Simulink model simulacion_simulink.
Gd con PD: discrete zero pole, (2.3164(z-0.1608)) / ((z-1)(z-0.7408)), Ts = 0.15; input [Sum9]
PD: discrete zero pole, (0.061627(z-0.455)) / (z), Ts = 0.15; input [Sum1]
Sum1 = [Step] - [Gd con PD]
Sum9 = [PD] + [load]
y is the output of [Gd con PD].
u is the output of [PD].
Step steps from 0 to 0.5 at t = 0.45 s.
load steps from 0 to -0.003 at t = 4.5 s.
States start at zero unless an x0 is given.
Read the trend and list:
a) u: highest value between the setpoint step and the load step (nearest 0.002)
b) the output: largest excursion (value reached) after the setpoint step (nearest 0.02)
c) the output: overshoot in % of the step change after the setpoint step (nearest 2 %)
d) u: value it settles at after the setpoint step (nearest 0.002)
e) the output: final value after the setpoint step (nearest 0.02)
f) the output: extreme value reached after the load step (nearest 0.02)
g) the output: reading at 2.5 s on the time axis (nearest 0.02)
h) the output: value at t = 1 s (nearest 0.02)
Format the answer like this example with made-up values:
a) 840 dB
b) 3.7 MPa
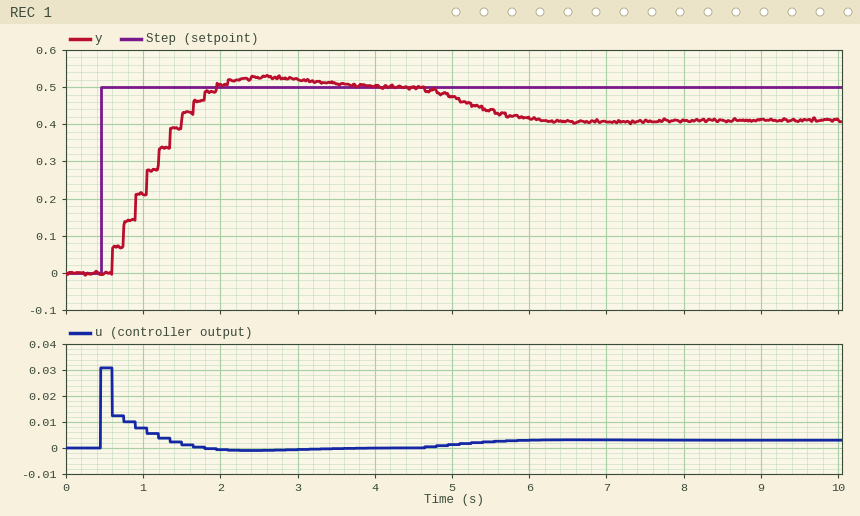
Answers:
a) 0.030
b) 0.52
c) 6 %
d) 0.000
e) 0.50
f) 0.40
g) 0.52
h) 0.22
